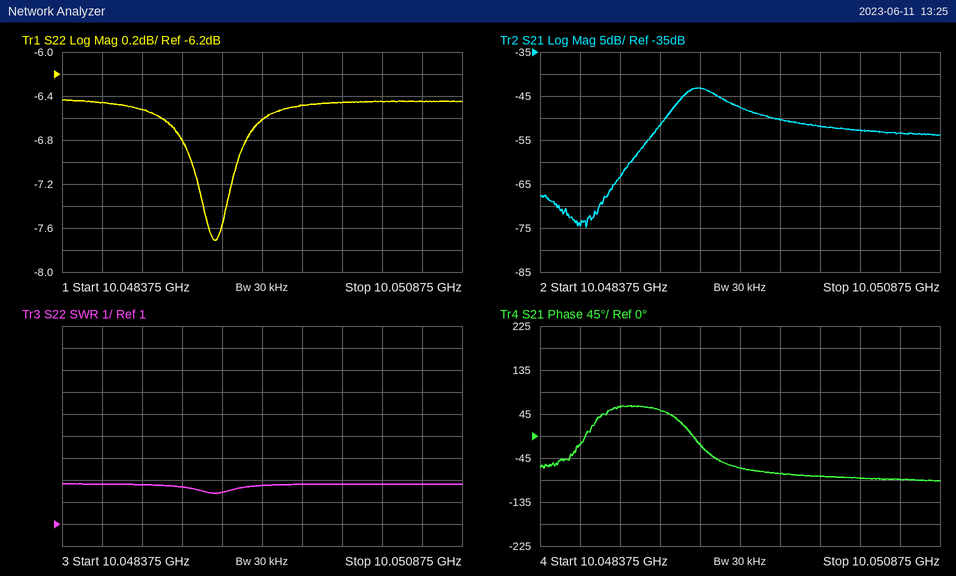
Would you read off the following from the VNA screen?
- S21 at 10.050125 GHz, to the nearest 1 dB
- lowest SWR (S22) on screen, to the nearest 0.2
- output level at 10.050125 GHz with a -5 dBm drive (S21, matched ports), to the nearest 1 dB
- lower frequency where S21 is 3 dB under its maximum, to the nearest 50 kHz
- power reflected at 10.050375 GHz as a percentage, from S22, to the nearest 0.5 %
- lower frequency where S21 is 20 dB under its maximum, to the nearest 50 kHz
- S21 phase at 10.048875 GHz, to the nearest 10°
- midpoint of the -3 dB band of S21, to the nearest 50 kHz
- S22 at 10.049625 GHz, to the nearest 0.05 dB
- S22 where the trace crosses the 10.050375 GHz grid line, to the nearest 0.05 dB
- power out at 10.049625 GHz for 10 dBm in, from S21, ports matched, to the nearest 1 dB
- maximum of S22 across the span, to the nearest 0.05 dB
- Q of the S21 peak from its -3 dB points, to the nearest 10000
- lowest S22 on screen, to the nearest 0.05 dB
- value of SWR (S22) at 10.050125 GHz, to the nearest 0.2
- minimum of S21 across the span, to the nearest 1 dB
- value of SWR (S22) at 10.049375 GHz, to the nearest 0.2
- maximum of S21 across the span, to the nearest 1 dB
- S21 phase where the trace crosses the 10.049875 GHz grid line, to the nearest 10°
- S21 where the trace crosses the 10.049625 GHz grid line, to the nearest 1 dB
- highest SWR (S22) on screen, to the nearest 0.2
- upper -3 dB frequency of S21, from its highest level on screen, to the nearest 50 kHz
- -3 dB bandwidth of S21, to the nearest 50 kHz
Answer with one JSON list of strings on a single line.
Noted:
["-52 dB", "2.4", "-57 dBm", "10.04925 GHz", "22.5 %", "10.04890 GHz", "60°", "10.04940 GHz", "-6.60 dB", "-6.45 dB", "-38 dBm", "-6.45 dB", "30000", "-7.70 dB", "2.8", "-75 dB", "2.4", "-43 dB", "-80°", "-48 dB", "2.8", "10.04955 GHz", "300 kHz"]
